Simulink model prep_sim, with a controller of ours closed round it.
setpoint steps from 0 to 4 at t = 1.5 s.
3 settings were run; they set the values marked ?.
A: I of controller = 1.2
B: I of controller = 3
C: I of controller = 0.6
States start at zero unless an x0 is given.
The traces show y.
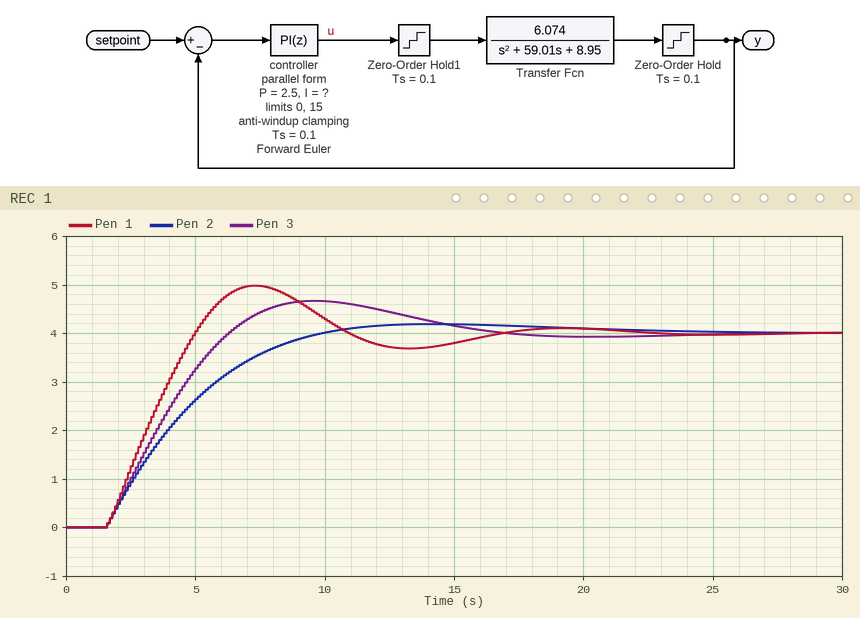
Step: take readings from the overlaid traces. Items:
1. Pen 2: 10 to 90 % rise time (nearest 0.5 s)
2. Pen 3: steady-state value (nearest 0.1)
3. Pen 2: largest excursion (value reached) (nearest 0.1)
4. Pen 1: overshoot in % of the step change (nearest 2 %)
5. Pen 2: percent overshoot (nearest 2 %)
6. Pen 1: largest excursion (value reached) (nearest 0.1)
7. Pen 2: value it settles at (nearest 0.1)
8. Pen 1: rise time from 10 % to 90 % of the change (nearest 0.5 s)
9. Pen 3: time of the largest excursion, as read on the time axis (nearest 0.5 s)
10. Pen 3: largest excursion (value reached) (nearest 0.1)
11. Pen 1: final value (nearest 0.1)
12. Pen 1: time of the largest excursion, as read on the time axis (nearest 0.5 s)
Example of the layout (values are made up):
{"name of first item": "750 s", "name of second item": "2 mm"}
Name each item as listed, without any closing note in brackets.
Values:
{"Pen 2: 10 to 90 % rise time": "5.5 s", "Pen 3: steady-state value": "4.0", "Pen 2: largest excursion (value reached)": "4.2", "Pen 1: overshoot in % of the step change": "24 %", "Pen 2: percent overshoot": "4 %", "Pen 1: largest excursion (value reached)": "5.0", "Pen 2: value it settles at": "4.0", "Pen 1: rise time from 10 % to 90 % of the change": "2.5 s", "Pen 3: time of the largest excursion, as read on the time axis": "9.5 s", "Pen 3: largest excursion (value reached)": "4.7", "Pen 1: final value": "4.0", "Pen 1: time of the largest excursion, as read on the time axis": "7.5 s"}
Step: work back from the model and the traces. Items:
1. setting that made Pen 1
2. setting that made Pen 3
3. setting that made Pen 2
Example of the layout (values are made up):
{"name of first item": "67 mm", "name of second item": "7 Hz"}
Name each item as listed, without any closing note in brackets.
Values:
{"setting that made Pen 1": "B", "setting that made Pen 3": "A", "setting that made Pen 2": "C"}
